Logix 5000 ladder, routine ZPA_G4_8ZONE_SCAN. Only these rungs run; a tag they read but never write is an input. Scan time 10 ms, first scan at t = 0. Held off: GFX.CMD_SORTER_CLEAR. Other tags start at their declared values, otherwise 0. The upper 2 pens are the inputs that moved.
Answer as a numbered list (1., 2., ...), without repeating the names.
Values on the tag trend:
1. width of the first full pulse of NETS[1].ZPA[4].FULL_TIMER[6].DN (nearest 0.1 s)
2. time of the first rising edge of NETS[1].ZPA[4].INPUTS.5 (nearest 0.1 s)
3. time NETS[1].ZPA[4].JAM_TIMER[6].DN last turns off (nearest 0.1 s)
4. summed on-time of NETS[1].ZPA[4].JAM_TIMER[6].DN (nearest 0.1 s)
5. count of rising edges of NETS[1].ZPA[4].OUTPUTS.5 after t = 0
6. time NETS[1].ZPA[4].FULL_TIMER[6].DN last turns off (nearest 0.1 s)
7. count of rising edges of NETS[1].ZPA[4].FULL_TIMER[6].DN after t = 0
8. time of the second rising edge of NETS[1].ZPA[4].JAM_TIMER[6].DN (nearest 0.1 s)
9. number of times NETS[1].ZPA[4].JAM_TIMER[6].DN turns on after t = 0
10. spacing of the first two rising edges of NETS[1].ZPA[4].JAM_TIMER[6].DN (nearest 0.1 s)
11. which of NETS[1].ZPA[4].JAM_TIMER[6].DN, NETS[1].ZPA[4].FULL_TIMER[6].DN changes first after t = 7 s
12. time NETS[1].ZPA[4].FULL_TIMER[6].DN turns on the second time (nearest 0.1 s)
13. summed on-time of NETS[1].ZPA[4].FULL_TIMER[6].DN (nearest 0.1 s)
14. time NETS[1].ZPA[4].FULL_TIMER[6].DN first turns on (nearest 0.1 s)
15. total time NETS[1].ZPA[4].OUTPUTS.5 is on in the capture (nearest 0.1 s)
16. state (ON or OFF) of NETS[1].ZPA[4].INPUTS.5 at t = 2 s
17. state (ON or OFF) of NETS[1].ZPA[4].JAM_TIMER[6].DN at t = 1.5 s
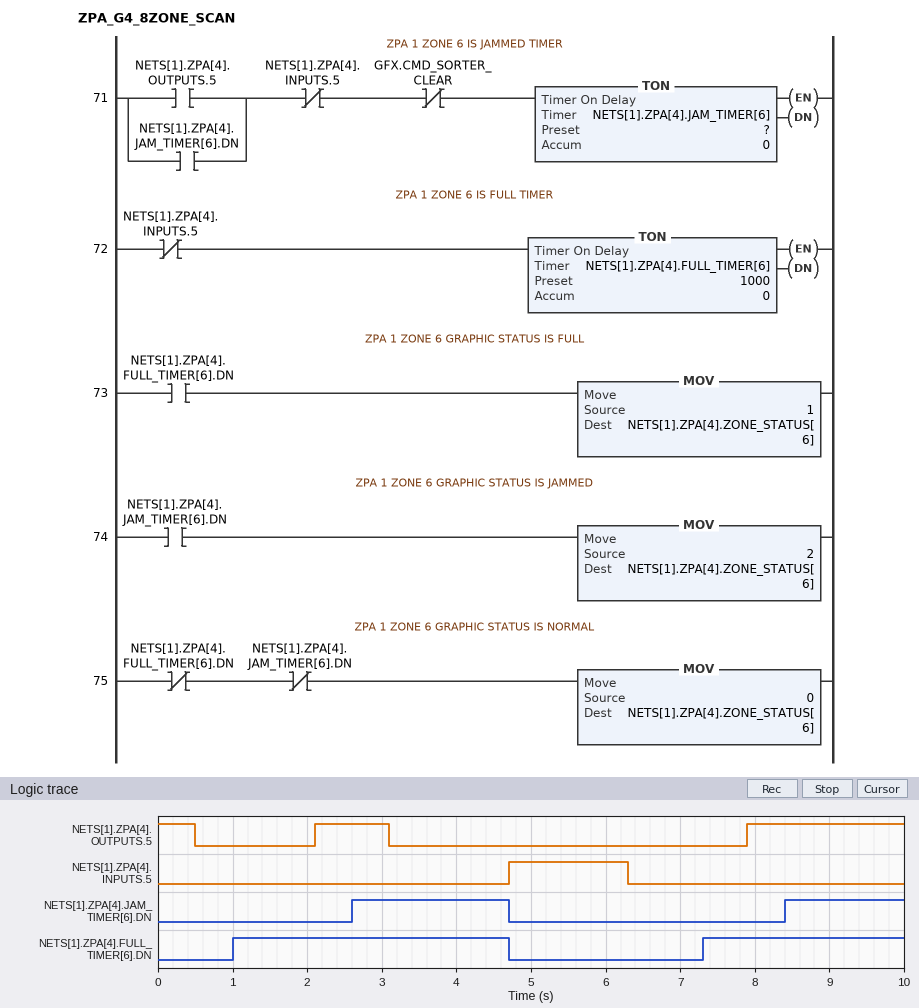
1. 3.7 s
2. 4.7 s
3. 4.7 s
4. 3.7 s
5. 2
6. 4.7 s
7. 2
8. 8.4 s
9. 2
10. 5.8 s
11. NETS[1].ZPA[4].FULL_TIMER[6].DN
12. 7.3 s
13. 6.4 s
14. 1.0 s
15. 3.6 s
16. OFF
17. OFF
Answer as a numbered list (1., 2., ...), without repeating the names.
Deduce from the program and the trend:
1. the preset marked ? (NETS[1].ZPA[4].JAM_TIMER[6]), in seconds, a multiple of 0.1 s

1. 0.5 s
